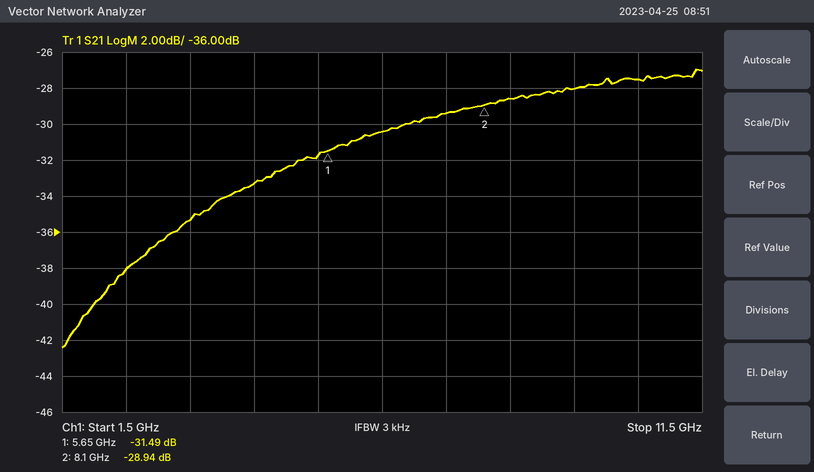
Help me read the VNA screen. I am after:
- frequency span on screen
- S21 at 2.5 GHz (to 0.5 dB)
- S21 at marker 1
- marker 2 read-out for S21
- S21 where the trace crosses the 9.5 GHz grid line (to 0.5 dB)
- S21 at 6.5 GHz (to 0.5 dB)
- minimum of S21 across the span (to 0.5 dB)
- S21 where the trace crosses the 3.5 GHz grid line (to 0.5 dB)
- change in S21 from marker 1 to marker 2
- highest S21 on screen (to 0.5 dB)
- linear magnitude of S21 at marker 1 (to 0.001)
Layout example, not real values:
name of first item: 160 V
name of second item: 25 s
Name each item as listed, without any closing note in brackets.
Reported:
frequency span on screen: 10 GHz
S21 at 2.5 GHz: -38.0 dB
S21 at marker 1: -31.49 dB
marker 2 read-out for S21: -28.94 dB
S21 where the trace crosses the 9.5 GHz grid line: -28.0 dB
S21 at 6.5 GHz: -30.5 dB
minimum of S21 across the span: -42.5 dB
S21 where the trace crosses the 3.5 GHz grid line: -35.5 dB
change in S21 from marker 1 to marker 2: 2.55 dB
highest S21 on screen: -27.0 dB
linear magnitude of S21 at marker 1: 0.027
